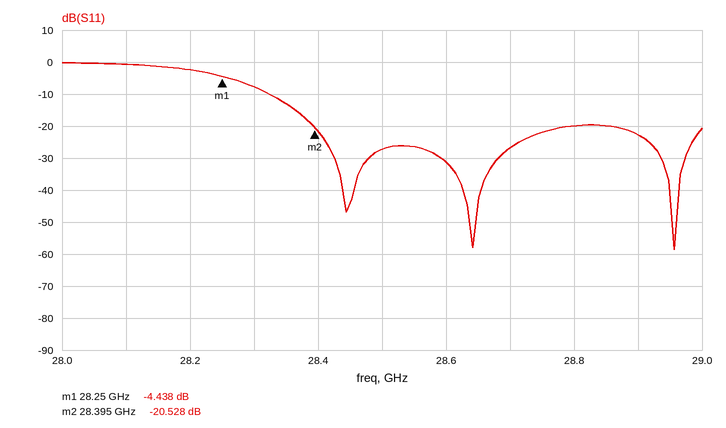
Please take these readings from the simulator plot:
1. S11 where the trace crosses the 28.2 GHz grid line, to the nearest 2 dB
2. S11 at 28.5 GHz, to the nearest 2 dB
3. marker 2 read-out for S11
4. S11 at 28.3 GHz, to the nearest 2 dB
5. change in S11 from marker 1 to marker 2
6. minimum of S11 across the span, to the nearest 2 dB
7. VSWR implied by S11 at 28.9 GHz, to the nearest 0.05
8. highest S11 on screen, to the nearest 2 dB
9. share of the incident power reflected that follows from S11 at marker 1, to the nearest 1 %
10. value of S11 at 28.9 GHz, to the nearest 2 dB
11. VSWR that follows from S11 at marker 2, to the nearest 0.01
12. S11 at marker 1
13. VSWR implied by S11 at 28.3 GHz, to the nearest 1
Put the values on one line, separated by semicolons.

-2 dB; -28 dB; -20.528 dB; -8 dB; -16.090 dB; -58 dB; 1.15; 0 dB; 36 %; -22 dB; 1.21; -4.438 dB; 2
